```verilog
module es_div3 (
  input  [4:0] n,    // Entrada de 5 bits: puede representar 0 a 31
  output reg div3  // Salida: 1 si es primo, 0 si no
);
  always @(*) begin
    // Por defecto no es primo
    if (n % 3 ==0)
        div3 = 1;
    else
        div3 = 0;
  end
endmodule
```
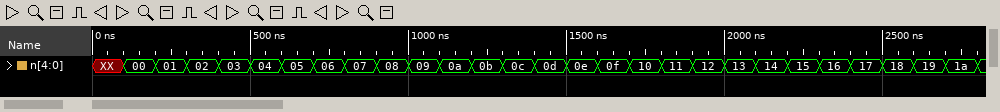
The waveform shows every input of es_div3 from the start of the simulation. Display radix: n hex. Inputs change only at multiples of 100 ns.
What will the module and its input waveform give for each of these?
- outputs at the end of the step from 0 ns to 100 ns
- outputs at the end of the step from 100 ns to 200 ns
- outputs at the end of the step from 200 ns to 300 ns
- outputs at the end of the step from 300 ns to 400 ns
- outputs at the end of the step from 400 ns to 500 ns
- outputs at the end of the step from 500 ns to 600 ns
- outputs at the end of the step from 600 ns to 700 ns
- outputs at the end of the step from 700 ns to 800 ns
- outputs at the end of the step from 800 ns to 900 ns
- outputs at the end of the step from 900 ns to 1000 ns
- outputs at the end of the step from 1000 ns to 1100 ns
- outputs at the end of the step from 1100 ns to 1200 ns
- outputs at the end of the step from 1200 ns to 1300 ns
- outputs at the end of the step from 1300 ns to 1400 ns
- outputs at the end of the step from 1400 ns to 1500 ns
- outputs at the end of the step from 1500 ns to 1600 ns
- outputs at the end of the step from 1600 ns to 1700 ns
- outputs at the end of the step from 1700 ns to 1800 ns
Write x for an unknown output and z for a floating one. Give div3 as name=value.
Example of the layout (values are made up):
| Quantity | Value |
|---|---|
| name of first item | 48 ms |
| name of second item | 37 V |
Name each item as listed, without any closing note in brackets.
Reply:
| Quantity | Value |
|---|---|
| outputs at the end of the step from 0 ns to 100 ns | div3=x |
| outputs at the end of the step from 100 ns to 200 ns | div3=1 |
| outputs at the end of the step from 200 ns to 300 ns | div3=0 |
| outputs at the end of the step from 300 ns to 400 ns | div3=0 |
| outputs at the end of the step from 400 ns to 500 ns | div3=1 |
| outputs at the end of the step from 500 ns to 600 ns | div3=0 |
| outputs at the end of the step from 600 ns to 700 ns | div3=0 |
| outputs at the end of the step from 700 ns to 800 ns | div3=1 |
| outputs at the end of the step from 800 ns to 900 ns | div3=0 |
| outputs at the end of the step from 900 ns to 1000 ns | div3=0 |
| outputs at the end of the step from 1000 ns to 1100 ns | div3=1 |
| outputs at the end of the step from 1100 ns to 1200 ns | div3=0 |
| outputs at the end of the step from 1200 ns to 1300 ns | div3=0 |
| outputs at the end of the step from 1300 ns to 1400 ns | div3=1 |
| outputs at the end of the step from 1400 ns to 1500 ns | div3=0 |
| outputs at the end of the step from 1500 ns to 1600 ns | div3=0 |
| outputs at the end of the step from 1600 ns to 1700 ns | div3=1 |
| outputs at the end of the step from 1700 ns to 1800 ns | div3=0 |
